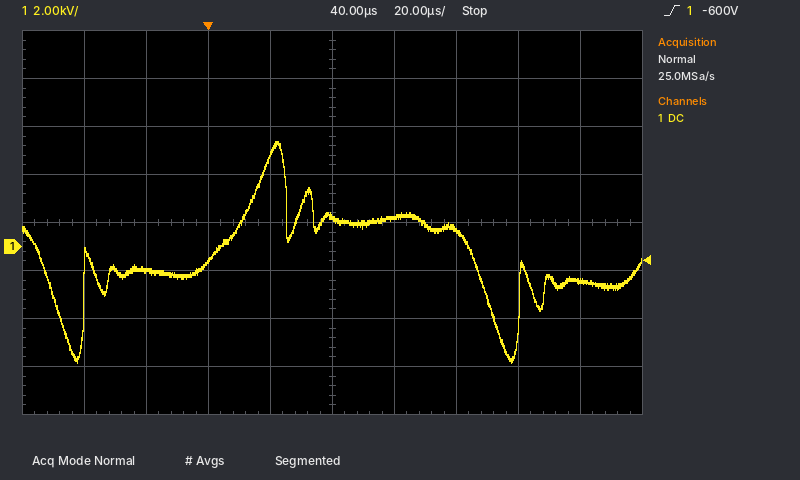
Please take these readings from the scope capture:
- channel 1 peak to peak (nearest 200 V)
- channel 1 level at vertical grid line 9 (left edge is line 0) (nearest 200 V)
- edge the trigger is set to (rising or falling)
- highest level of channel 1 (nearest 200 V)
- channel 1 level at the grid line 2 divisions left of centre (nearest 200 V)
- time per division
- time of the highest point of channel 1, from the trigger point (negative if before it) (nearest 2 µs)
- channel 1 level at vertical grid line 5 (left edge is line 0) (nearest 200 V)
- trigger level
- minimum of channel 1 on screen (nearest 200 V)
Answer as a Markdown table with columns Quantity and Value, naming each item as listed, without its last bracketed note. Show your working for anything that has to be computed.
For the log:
| Quantity | Value |
|---|---|
| channel 1 peak to peak | 4.4 kV − (-4.8 kV) = 9.2 kV |
| channel 1 level at vertical grid line 9 (left edge is line 0) | -1.4 kV |
| edge the trigger is set to | rising |
| highest level of channel 1 | 4.4 kV |
| channel 1 level at the grid line 2 divisions left of centre | -600 V |
| time per division | 20 µs |
| time of the highest point of channel 1, from the trigger point (negative if before it) | +22 µs |
| channel 1 level at vertical grid line 5 (left edge is line 0) | 1.2 kV |
| trigger level | -600 V |
| minimum of channel 1 on screen | -4.8 kV |
